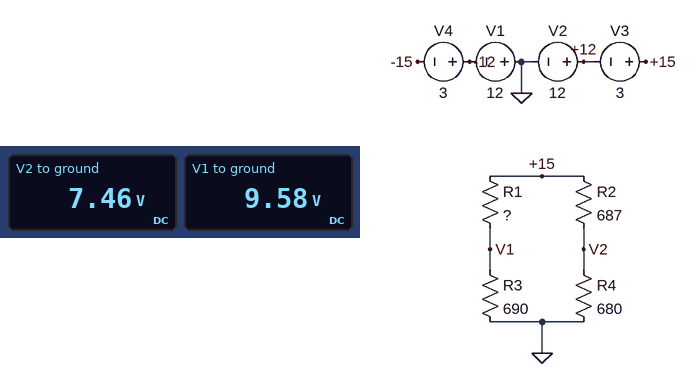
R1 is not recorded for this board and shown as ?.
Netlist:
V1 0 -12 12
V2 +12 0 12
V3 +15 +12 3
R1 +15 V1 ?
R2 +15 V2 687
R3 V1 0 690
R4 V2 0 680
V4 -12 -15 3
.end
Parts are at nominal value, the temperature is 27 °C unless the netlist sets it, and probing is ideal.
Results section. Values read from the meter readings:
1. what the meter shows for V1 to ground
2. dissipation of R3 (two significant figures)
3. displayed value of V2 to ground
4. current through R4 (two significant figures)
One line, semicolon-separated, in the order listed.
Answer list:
9.58 V; 130 mW; 7.46 V; 11 mA
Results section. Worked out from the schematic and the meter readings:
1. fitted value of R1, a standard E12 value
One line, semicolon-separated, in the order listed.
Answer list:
390 Ω
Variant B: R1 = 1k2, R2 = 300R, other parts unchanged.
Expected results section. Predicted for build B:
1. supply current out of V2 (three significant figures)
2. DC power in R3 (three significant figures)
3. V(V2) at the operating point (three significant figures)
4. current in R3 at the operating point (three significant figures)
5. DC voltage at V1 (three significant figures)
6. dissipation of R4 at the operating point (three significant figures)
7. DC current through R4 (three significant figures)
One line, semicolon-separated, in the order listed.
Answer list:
23.2 mA; 43.5 mW; 10.4 V; 7.94 mA; 5.48 V; 159 mW; 15.3 mA
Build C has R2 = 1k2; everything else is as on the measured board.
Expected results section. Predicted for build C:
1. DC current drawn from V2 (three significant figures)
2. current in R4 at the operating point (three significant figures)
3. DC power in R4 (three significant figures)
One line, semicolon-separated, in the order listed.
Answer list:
21.9 mA; 7.98 mA; 43.3 mW
